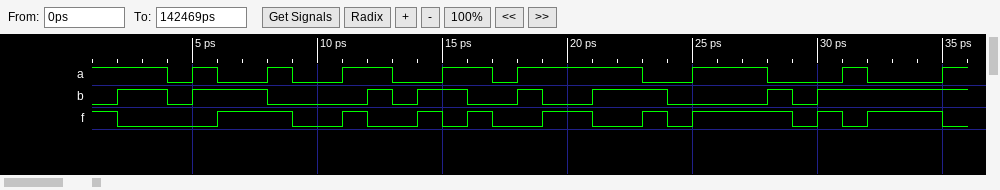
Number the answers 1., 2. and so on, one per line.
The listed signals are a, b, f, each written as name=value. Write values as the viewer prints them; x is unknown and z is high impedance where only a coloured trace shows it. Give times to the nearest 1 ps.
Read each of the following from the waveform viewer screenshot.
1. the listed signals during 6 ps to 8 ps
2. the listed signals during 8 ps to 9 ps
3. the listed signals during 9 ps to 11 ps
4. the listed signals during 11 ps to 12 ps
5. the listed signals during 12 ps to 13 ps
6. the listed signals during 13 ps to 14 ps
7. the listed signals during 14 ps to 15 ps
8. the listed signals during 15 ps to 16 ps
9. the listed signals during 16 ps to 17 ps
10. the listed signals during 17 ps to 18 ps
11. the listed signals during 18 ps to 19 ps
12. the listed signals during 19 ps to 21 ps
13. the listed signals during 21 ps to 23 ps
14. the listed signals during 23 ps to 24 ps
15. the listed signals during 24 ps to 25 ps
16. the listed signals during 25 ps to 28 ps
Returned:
1. a=0, b=1, f=1
2. a=1, b=0, f=1
3. a=0, b=0, f=0
4. a=1, b=0, f=1
5. a=1, b=1, f=0
6. a=0, b=0, f=0
7. a=0, b=1, f=1
8. a=1, b=1, f=0
9. a=1, b=0, f=1
10. a=0, b=0, f=0
11. a=1, b=1, f=0
12. a=1, b=0, f=1
13. a=1, b=1, f=0
14. a=0, b=1, f=1
15. a=0, b=0, f=0
16. a=1, b=0, f=1
